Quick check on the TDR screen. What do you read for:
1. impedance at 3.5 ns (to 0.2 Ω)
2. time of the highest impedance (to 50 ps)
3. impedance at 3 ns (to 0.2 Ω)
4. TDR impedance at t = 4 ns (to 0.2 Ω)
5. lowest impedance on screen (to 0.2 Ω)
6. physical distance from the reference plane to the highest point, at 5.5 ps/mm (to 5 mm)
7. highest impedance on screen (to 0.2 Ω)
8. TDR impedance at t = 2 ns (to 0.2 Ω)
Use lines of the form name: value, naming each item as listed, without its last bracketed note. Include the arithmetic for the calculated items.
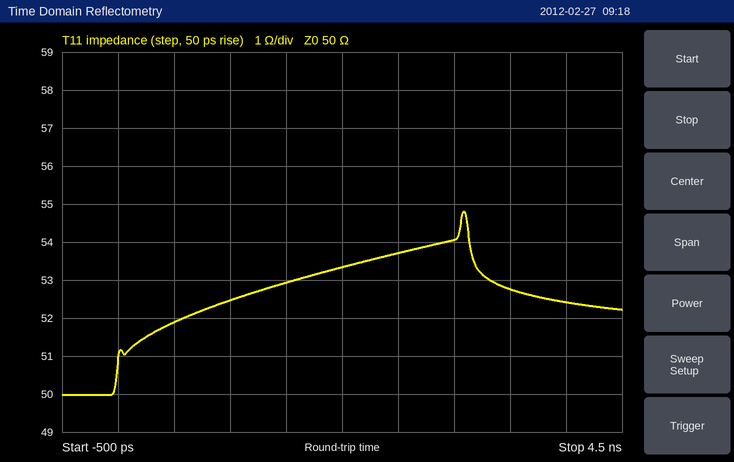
impedance at 3.5 ns: 52.8 Ω
time of the highest impedance: 3.10 ns
impedance at 3 ns: 54.0 Ω
TDR impedance at t = 4 ns: 52.4 Ω
lowest impedance on screen: 50.0 Ω
physical distance from the reference plane to the highest point, at 5.5 ps/mm: 3.10 ns / 2 / 5.5 ps/mm ≈ 282 mm, so 280 mm to the nearest 5 mm
highest impedance on screen: 54.8 Ω
TDR impedance at t = 2 ns: 53.4 Ω
